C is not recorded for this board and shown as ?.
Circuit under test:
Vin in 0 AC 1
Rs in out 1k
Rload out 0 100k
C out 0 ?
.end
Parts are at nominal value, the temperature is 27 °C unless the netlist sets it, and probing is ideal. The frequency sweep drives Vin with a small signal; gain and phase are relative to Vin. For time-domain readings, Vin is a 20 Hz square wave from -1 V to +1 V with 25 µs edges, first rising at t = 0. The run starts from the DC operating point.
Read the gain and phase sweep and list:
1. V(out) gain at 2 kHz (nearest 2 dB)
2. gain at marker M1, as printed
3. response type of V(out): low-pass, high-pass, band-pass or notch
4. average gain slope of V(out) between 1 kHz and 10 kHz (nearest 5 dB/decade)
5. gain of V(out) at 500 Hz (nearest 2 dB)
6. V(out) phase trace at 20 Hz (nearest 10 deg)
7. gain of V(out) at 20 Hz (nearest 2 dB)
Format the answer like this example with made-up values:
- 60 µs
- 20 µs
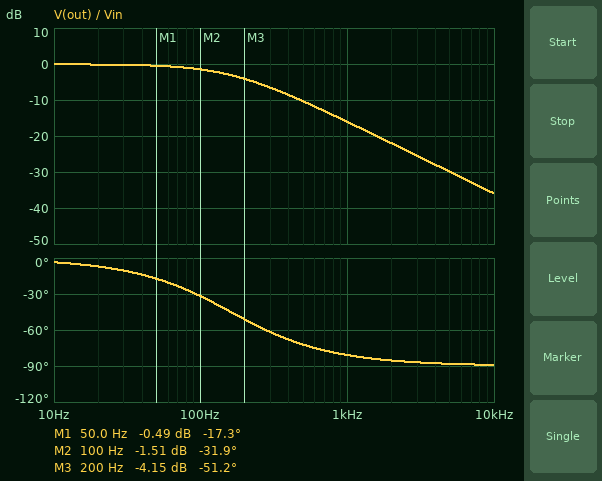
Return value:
- -22 dB
- -0.49 dB
- low-pass
- -20 dB/decade
- -10 dB
- -10 deg
- 0 dB
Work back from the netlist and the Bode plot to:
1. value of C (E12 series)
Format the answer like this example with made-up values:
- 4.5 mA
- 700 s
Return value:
- 1 µF
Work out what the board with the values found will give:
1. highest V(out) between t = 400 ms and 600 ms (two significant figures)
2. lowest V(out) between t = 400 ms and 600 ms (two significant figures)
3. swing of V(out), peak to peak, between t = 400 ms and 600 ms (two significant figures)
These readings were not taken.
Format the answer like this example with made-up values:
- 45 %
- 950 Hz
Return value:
- 990 mV
- -990 mV
- 2.0 V
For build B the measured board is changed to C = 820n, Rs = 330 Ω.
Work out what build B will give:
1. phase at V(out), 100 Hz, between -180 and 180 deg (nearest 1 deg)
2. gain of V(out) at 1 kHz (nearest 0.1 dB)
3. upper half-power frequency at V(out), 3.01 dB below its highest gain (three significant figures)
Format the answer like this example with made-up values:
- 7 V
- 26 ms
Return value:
- -10 deg
- -5.9 dB
- 590 Hz
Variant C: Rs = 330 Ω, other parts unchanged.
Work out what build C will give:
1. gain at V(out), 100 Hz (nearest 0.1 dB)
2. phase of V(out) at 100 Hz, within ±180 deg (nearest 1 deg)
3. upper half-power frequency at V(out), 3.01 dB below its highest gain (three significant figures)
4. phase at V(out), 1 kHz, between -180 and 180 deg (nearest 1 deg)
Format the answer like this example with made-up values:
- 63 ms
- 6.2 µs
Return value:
- -0.2 dB
- -12 deg
- 484 Hz
- -64 deg
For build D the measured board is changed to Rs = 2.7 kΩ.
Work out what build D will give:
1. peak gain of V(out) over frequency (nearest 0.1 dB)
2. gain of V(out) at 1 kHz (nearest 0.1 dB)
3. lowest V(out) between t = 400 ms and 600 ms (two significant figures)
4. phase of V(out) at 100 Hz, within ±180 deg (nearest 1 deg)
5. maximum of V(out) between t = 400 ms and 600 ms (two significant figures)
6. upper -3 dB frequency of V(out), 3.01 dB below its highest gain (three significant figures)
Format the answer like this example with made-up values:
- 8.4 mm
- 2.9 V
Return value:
- -0.2 dB
- -24.6 dB
- -970 mV
- -59 deg
- 970 mV
- 60.5 Hz
